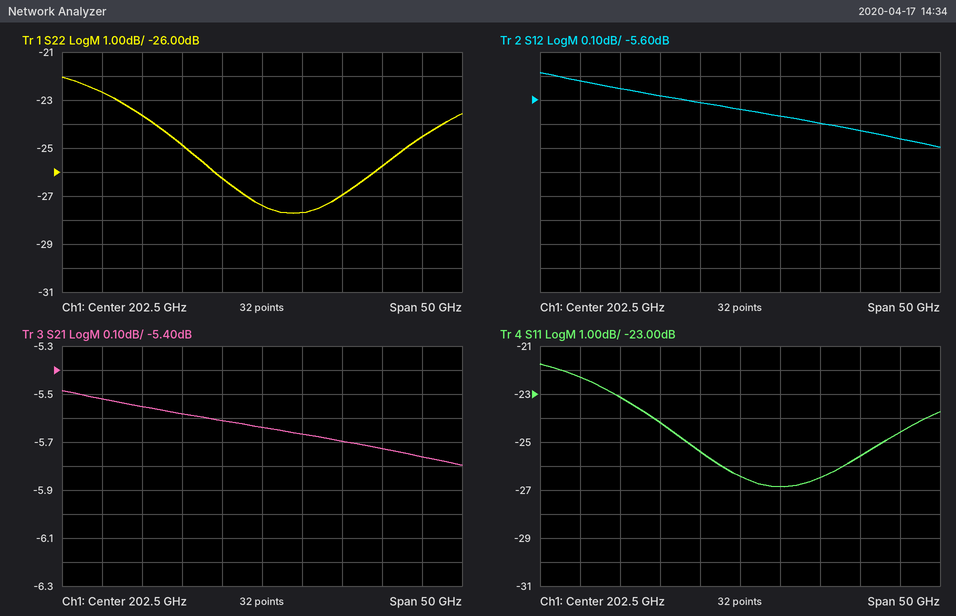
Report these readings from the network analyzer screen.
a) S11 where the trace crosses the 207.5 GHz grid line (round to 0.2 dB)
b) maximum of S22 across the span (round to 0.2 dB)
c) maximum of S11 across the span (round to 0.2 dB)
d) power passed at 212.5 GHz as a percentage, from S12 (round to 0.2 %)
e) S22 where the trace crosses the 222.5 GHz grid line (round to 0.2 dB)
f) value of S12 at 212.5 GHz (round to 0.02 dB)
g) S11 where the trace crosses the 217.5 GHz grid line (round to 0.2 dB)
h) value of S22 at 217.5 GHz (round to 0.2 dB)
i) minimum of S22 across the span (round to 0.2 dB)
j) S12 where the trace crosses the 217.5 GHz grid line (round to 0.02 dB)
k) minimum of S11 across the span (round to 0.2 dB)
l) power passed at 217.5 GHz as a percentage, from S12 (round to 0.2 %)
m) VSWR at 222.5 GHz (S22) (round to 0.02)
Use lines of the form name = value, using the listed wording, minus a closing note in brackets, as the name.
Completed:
S11 where the trace crosses the 207.5 GHz grid line = -26.8 dB
maximum of S22 across the span = -22.0 dB
maximum of S11 across the span = -21.8 dB
power passed at 212.5 GHz as a percentage, from S12 = 27.0 %
S22 where the trace crosses the 222.5 GHz grid line = -24.6 dB
value of S12 at 212.5 GHz = -5.70 dB
S11 where the trace crosses the 217.5 GHz grid line = -25.6 dB
value of S22 at 217.5 GHz = -25.8 dB
minimum of S22 across the span = -27.8 dB
S12 where the trace crosses the 217.5 GHz grid line = -5.72 dB
minimum of S11 across the span = -26.8 dB
power passed at 217.5 GHz as a percentage, from S12 = 26.8 %
VSWR at 222.5 GHz (S22) = 1.12
